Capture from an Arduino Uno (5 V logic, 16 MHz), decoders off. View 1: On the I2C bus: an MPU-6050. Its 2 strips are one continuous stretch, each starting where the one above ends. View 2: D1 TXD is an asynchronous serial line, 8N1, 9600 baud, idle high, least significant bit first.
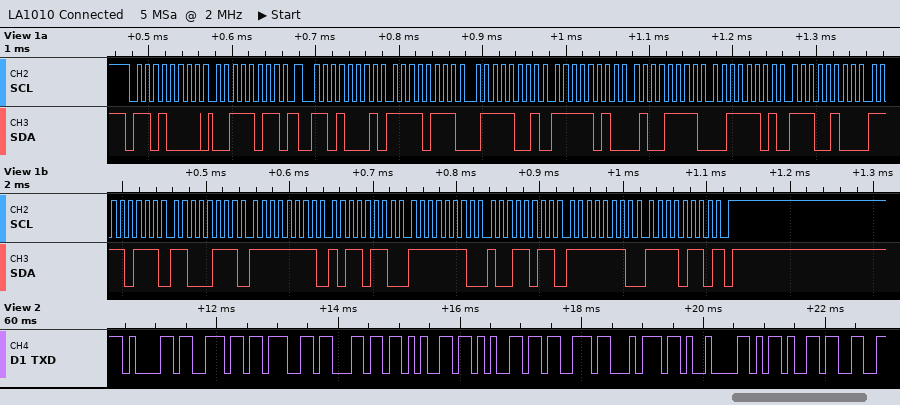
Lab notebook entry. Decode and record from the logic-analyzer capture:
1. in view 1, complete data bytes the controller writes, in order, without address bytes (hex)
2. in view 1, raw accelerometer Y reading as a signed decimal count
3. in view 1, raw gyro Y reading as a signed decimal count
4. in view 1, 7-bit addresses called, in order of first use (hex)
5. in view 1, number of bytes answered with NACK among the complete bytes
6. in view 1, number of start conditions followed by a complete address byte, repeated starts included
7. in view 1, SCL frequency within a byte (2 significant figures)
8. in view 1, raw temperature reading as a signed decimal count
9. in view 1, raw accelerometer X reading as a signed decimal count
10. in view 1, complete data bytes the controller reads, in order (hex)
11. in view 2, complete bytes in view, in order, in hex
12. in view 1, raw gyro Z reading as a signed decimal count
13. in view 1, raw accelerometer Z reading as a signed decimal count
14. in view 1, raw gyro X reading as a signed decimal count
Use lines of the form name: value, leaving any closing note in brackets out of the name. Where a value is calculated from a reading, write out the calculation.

in view 1, complete data bytes the controller writes, in order, without address bytes: 3B
in view 1, raw accelerometer Y reading as a signed decimal count: 0xFA4F = -1457
in view 1, raw gyro Y reading as a signed decimal count: 0xFE9B = -357
in view 1, 7-bit addresses called, in order of first use: 0x68
in view 1, number of bytes answered with NACK among the complete bytes: 1
in view 1, number of start conditions followed by a complete address byte, repeated starts included: 2
in view 1, SCL frequency within a byte: 100 kHz
in view 1, raw temperature reading as a signed decimal count: 0xF7C7 = -2105
in view 1, raw accelerometer X reading as a signed decimal count: 0xF779 = -2183
in view 1, complete data bytes the controller reads, in order: F7 79 FA 4F 3D E4 F7 C7 FF B6 FE 9B FE F6
in view 2, complete bytes in view, in order, in hex: 61 6E 67 6C 65 65 73 74 09 2D 33
in view 1, raw gyro Z reading as a signed decimal count: 0xFEF6 = -266
in view 1, raw accelerometer Z reading as a signed decimal count: 0x3DE4 = 15844
in view 1, raw gyro X reading as a signed decimal count: 0xFFB6 = -74
